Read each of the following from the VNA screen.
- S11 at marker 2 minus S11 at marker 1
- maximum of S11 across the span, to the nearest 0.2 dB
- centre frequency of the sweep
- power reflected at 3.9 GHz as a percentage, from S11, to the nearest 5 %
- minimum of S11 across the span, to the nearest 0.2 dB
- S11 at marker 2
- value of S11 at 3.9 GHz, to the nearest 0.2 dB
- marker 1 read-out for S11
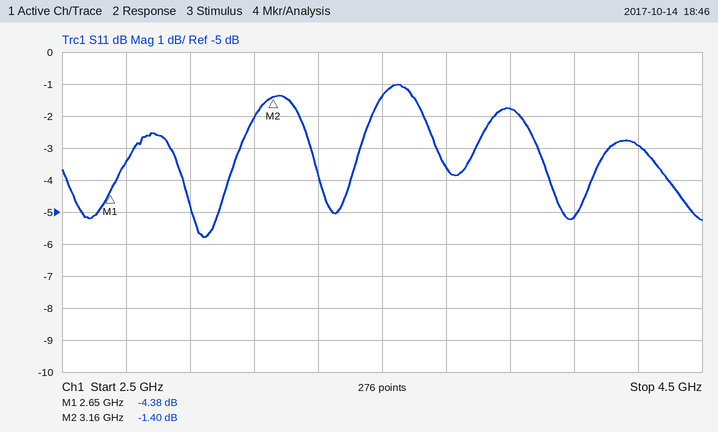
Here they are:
2.98 dB
-1.0 dB
3.5 GHz
65 %
-5.8 dB
-1.40 dB
-1.8 dB
-4.38 dB
